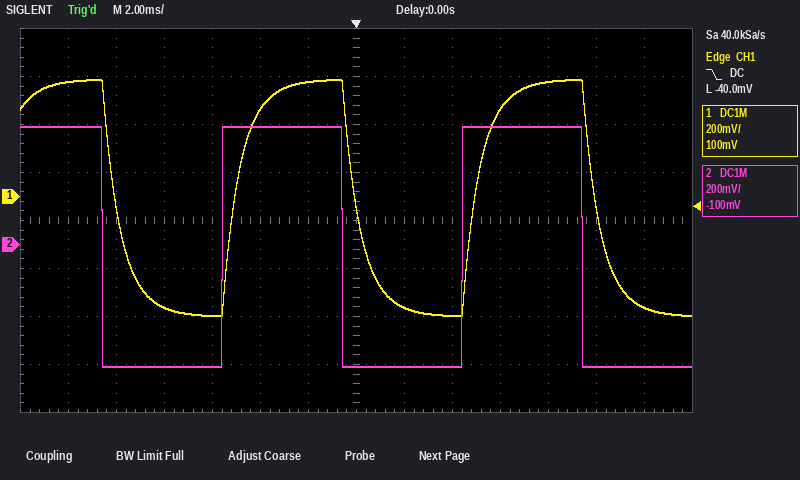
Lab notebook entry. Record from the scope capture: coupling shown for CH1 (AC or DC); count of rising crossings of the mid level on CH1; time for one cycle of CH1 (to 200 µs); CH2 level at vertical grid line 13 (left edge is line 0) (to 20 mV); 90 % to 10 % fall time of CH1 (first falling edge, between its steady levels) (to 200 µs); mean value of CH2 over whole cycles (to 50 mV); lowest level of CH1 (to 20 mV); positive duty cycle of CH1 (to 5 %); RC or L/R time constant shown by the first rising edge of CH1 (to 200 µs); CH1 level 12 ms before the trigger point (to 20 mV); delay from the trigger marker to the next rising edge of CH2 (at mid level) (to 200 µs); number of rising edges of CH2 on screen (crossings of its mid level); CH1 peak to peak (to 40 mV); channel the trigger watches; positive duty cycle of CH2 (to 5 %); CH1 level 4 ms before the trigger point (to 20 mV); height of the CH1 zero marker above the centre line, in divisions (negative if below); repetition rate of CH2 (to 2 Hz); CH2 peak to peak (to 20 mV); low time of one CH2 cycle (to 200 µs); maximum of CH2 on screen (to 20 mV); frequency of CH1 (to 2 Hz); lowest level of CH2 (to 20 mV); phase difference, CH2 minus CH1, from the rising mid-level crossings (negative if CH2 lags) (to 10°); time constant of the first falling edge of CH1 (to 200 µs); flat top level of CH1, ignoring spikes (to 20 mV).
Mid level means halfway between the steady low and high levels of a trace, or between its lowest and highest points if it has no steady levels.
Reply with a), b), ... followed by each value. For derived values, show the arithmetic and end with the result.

a) DC
b) 2
c) 10.0 ms
d) -500 mV
e) 1.6 ms
f) -500 mV + 0.5 × (500 mV − (-500 mV)) ≈ 0 mV
g) -500 mV
h) 50 %
i) 1.6 ms / 2.2 ≈ 727 µs, so 800 µs to the nearest 200 µs
j) 480 mV
k) 4.4 ms
l) 2
m) 1.00 V
n) CH1
o) 5.0 ms / 10.0 ms ≈ 50 %
p) 360 mV
q) +0.5 div
r) 1 / 10.0 ms ≈ 100 Hz
s) 500 mV − (-500 mV) = 1.00 V
t) 5.0 ms
u) 500 mV
v) 1 / 10.0 ms ≈ 100 Hz
w) -500 mV
x) +20°
y) 1.6 ms / 2.2 ≈ 727 µs, so 800 µs to the nearest 200 µs
z) 480 mV
